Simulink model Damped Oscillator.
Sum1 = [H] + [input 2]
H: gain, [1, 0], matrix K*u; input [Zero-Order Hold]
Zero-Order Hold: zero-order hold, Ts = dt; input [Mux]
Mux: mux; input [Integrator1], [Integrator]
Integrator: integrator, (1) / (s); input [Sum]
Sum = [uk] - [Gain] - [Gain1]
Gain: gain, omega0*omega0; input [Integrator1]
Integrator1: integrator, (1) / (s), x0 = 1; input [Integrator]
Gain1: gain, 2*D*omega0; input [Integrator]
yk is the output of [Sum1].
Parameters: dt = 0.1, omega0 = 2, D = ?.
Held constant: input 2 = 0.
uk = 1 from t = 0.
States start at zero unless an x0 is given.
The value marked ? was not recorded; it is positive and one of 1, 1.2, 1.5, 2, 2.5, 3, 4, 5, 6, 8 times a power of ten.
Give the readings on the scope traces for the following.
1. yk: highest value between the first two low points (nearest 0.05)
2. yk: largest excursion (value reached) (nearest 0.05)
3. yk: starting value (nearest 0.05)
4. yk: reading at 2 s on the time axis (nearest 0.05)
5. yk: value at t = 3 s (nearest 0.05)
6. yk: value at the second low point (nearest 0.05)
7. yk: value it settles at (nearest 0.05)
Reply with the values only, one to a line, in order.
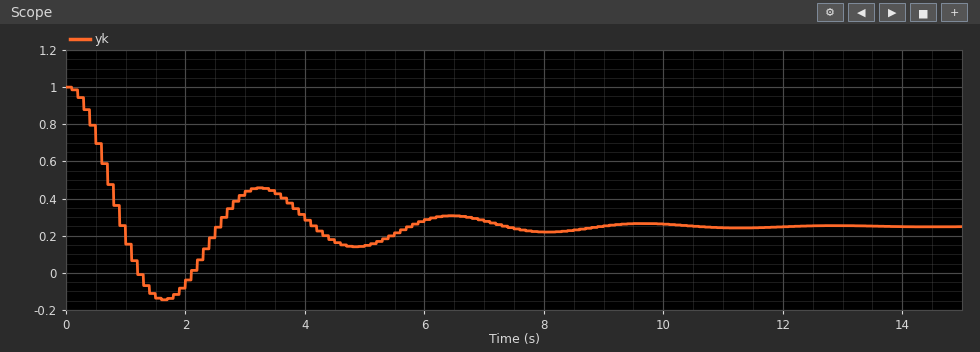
0.45
-0.15
1.00
-0.05
0.45
0.15
0.25
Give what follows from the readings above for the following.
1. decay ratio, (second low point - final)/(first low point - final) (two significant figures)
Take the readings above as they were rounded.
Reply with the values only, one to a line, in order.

0.25
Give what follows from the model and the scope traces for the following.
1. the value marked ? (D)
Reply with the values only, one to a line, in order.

0.2
